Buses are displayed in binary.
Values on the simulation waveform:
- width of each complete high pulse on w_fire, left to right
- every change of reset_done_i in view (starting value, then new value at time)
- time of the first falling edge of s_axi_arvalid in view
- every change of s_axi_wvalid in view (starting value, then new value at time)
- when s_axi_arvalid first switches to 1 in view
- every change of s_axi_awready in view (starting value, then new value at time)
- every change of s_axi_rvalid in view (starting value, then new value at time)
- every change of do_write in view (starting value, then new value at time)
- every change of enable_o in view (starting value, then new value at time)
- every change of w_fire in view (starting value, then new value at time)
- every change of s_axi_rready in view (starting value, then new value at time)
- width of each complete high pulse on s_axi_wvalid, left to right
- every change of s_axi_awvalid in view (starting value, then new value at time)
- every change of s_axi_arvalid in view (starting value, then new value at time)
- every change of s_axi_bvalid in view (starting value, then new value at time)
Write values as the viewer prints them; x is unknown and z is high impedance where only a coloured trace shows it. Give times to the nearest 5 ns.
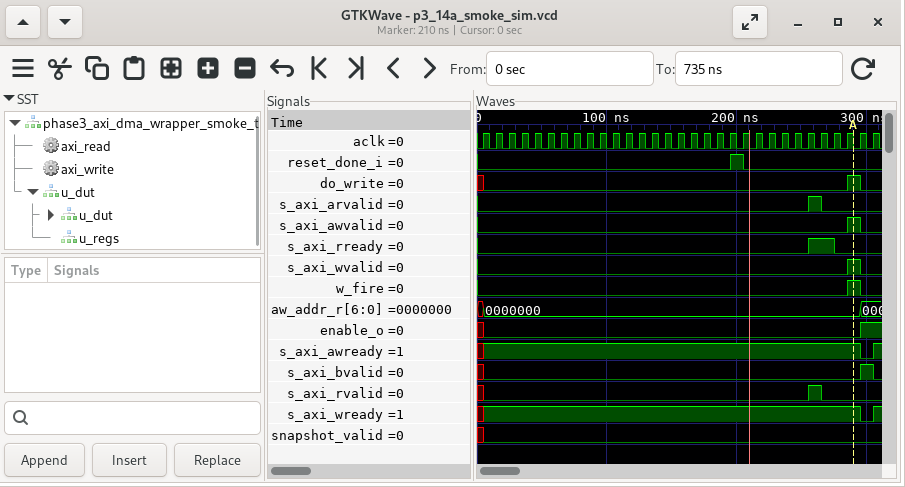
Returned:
10 ns
0, 1 at 195 ns, 0 at 205 ns
265 ns
0, 1 at 285 ns, 0 at 295 ns
255 ns
x, 1 at 5 ns, 0 at 295 ns, 1 at 305 ns
x, 0 at 5 ns, 1 at 255 ns, 0 at 265 ns
x, 0 at 5 ns, 1 at 285 ns, 0 at 295 ns
x, 0 at 5 ns, 1 at 295 ns
0, 1 at 285 ns, 0 at 295 ns
0, 1 at 255 ns, 0 at 275 ns
10 ns
0, 1 at 285 ns, 0 at 295 ns
0, 1 at 255 ns, 0 at 265 ns
x, 0 at 5 ns, 1 at 295 ns, 0 at 305 ns
